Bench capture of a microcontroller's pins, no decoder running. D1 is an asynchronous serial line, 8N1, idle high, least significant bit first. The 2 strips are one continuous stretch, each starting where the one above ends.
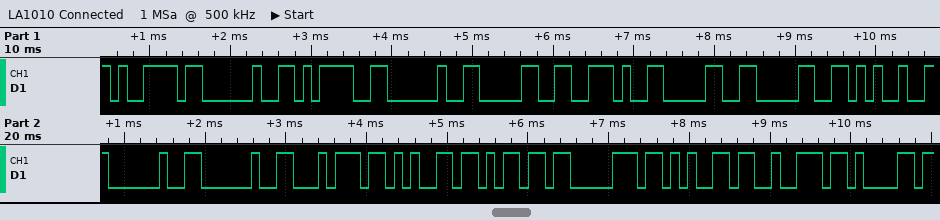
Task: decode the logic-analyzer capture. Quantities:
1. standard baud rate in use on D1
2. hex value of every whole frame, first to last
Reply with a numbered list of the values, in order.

1. 9600 baud
2. 0x79 0x20 0x3D 0x20 0x30 0x2E 0x30 0x30 0x25 0x20 0x20 0x74 0x65 0x6D 0x70 0x65 0x72 0x61
